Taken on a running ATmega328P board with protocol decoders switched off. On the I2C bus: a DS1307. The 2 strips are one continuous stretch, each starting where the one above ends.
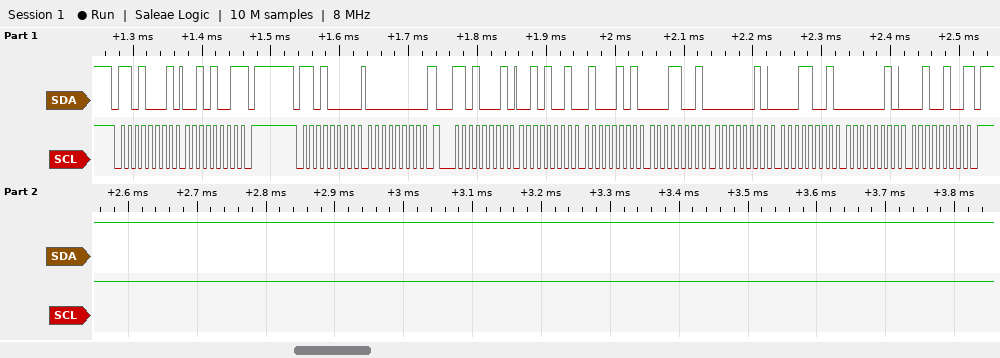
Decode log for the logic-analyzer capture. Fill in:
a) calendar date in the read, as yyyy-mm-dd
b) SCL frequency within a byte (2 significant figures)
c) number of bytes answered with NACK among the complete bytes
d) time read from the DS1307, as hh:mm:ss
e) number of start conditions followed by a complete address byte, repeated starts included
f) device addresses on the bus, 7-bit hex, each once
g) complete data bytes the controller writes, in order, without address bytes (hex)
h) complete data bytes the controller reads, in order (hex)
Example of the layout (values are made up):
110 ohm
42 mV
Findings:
2024-02-19
100 kHz
2
19:45:29
3
0x68
00
29 29 45 19 02 19 02 24
